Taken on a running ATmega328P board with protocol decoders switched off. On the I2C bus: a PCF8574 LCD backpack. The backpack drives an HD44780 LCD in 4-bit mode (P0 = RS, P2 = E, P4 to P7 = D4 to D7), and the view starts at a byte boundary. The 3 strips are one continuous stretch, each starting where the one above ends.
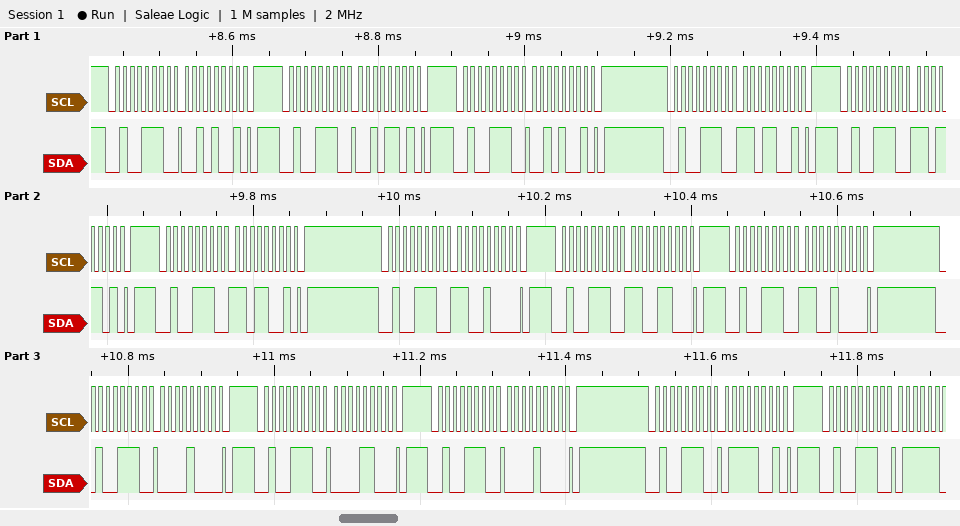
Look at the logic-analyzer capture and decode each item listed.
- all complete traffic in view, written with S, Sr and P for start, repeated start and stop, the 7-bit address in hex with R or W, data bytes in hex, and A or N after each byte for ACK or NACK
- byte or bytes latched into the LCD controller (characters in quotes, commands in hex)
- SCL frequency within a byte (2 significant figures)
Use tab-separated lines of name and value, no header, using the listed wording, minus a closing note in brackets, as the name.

all complete traffic in view, written with S, Sr and P for start, repeated start and stop, the 7-bit address in hex with R or W, data bytes in hex, and A or N after each byte for ACK or NACK	S 27W A 29 A P S 27W A 2D A P S 27W A 29 A P S 27W A D9 A P S 27W A DD A P S 27W A D9 A P S 27W A C8 A P S 27W A CC A P S 27W A C8 A P S 27W A 08 A P S 27W A 0C A P S 27W A 08 A P S 27W A 79 A P S 27W A
byte or bytes latched into the LCD controller	'-' 0xC0
SCL frequency within a byte	100 kHz
